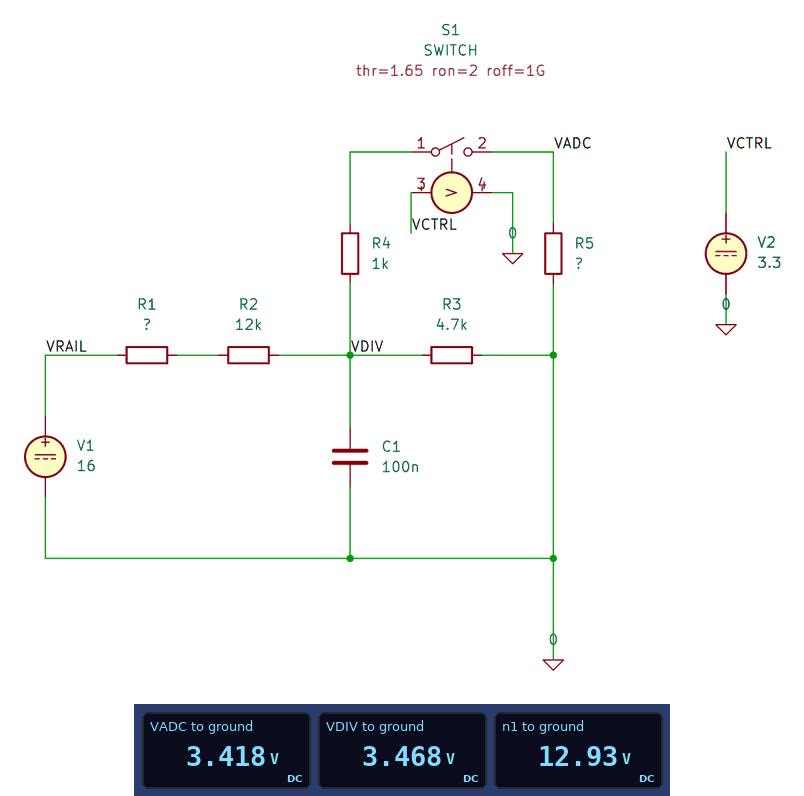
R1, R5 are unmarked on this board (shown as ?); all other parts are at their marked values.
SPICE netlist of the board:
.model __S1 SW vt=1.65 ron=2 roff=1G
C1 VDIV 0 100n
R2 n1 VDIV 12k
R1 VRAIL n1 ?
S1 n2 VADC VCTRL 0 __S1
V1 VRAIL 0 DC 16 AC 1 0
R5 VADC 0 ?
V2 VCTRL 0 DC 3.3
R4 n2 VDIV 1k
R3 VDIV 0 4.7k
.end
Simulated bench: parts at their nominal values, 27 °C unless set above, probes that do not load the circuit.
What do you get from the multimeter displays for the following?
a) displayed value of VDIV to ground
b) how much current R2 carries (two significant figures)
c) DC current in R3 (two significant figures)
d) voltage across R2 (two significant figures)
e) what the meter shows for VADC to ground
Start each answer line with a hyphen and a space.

- 3.468 V
- 790 µA
- 740 µA
- 9.5 V
- 3.418 V
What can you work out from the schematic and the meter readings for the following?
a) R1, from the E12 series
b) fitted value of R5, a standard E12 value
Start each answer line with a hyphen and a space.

- 3.9 kΩ
- 68 kΩ
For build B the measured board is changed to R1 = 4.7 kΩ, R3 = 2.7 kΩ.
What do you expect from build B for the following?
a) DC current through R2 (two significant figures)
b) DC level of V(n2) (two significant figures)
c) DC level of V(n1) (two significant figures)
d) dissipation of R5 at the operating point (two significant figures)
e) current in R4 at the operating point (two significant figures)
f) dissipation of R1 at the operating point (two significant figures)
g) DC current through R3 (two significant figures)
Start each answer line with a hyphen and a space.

- 830 µA
- 2.1 V
- 12 V
- 66 µW
- 31 µA
- 3.2 mW
- 800 µA
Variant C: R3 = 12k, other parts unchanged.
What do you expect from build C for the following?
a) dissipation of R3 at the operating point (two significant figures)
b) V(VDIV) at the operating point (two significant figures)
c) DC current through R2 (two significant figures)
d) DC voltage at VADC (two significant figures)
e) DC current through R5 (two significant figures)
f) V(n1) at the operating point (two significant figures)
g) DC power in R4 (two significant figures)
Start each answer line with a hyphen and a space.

- 3.3 mW
- 6.3 V
- 610 µA
- 6.2 V
- 91 µA
- 14 V
- 8.2 µW
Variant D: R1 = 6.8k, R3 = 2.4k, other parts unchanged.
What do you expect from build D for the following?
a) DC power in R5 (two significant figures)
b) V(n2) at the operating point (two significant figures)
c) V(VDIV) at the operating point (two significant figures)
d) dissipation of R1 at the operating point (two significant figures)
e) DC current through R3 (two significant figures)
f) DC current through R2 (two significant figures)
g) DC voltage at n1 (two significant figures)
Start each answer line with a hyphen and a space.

- 44 µW
- 1.7 V
- 1.8 V
- 3.9 mW
- 730 µA
- 760 µA
- 11 V
